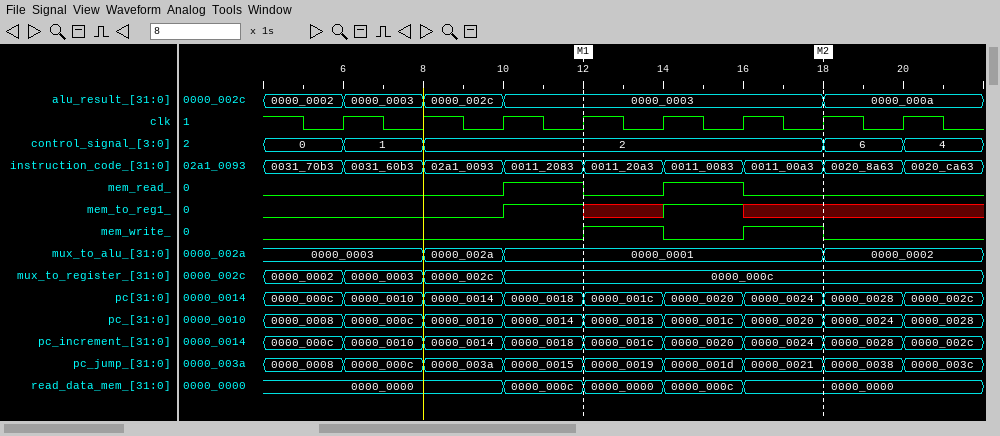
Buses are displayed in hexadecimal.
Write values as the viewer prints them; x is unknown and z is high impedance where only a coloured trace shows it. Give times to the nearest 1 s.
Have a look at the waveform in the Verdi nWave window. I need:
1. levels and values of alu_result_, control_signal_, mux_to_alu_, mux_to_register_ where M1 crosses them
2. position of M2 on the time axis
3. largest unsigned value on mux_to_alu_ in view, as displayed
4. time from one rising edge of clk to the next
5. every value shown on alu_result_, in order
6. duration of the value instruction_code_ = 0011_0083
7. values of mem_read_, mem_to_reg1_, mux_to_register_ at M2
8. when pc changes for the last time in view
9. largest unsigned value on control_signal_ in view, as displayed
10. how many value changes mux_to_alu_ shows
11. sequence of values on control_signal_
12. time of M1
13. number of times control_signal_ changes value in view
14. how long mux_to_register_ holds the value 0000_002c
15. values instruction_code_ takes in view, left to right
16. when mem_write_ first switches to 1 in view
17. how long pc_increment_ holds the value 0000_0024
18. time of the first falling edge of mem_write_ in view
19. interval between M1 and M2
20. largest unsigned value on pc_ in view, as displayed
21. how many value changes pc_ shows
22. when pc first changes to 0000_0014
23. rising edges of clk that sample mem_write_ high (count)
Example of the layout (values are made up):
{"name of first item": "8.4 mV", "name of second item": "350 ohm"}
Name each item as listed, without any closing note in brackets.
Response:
{"levels and values of alu_result_, control_signal_, mux_to_alu_, mux_to_register_ where M1 crosses them": "alu_result_=0000_0003, control_signal_=2, mux_to_alu_=0000_0001, mux_to_register_=0000_000c", "position of M2 on the time axis": "18 s", "largest unsigned value on mux_to_alu_ in view, as displayed": "0000_002a", "time from one rising edge of clk to the next": "2 s", "every value shown on alu_result_, in order": "0000_0002, 0000_0003, 0000_002c, 0000_0003, 0000_000a", "duration of the value instruction_code_ = 0011_0083": "2 s", "values of mem_read_, mem_to_reg1_, mux_to_register_ at M2": "mem_read_=0, mem_to_reg1_=x, mux_to_register_=0000_000c", "when pc changes for the last time in view": "20 s", "largest unsigned value on control_signal_ in view, as displayed": "6", "how many value changes mux_to_alu_ shows": "3", "sequence of values on control_signal_": "0, 1, 2, 6, 4", "time of M1": "12 s", "number of times control_signal_ changes value in view": "4", "how long mux_to_register_ holds the value 0000_002c": "2 s", "values instruction_code_ takes in view, left to right": "0031_70b3, 0031_60b3, 02a1_0093, 0011_2083, 0011_20a3, 0011_0083, 0011_00a3, 0020_8a63, 0020_ca63", "when mem_write_ first switches to 1 in view": "12 s", "how long pc_increment_ holds the value 0000_0024": "2 s", "time of the first falling edge of mem_write_ in view": "14 s", "interval between M1 and M2": "6 s", "largest unsigned value on pc_ in view, as displayed": "0000_0028", "how many value changes pc_ shows": "8", "when pc first changes to 0000_0014": "8 s", "rising edges of clk that sample mem_write_ high": "2"}
